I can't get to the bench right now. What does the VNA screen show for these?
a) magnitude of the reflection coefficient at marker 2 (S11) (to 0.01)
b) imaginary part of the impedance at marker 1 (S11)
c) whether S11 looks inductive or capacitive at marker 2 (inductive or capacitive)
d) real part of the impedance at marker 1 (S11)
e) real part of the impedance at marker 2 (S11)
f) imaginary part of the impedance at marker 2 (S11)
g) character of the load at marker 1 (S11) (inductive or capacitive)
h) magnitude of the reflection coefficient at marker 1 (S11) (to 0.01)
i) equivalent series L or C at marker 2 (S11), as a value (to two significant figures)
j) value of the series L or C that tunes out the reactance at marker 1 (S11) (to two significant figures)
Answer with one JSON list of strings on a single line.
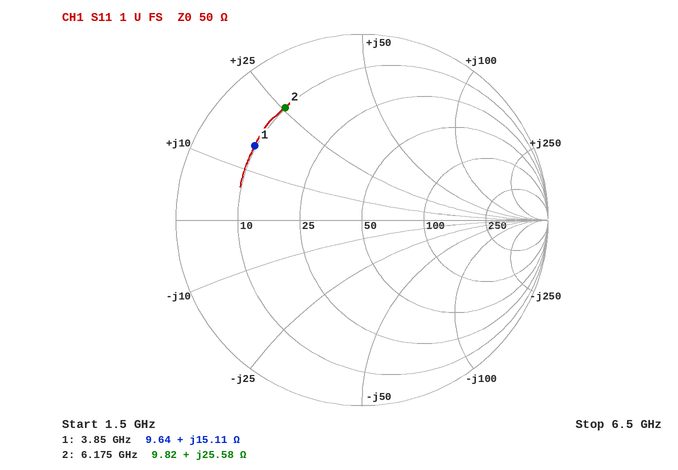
["0.73", "+15.11 Ω", "inductive", "9.64 Ω", "9.82 Ω", "+25.58 Ω", "inductive", "0.70", "660 pH", "2.7 pF"]
